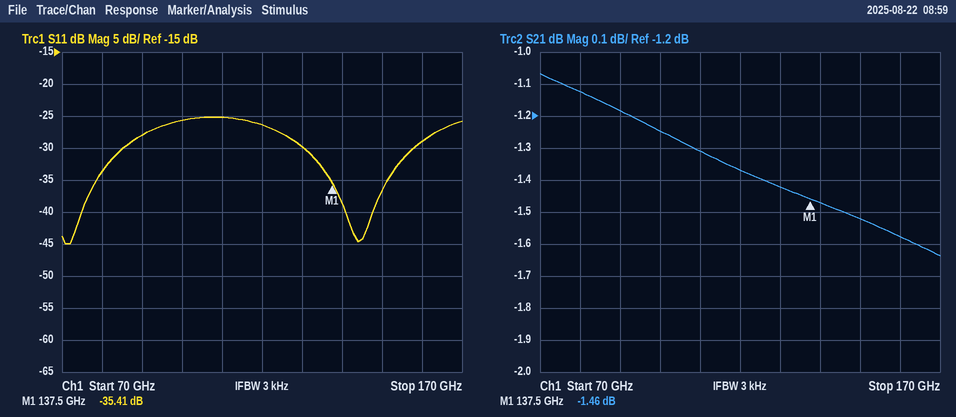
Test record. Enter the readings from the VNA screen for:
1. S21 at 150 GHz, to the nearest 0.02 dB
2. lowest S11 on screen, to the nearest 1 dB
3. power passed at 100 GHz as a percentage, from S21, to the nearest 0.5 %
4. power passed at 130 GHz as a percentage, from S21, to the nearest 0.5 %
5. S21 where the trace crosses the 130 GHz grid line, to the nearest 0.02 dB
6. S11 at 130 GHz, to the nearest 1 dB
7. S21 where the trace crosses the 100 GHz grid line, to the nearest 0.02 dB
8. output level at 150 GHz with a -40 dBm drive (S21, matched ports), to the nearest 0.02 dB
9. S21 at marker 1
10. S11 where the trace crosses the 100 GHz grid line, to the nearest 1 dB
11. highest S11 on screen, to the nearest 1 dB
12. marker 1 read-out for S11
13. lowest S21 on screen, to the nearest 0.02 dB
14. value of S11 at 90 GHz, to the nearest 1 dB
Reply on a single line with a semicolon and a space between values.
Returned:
-1.52 dB; -45 dB; 75.0 %; 72.0 %; -1.42 dB; -30 dB; -1.24 dB; -41.52 dBm; -1.46 dB; -26 dB; -25 dB; -35.41 dB; -1.64 dB; -28 dB
